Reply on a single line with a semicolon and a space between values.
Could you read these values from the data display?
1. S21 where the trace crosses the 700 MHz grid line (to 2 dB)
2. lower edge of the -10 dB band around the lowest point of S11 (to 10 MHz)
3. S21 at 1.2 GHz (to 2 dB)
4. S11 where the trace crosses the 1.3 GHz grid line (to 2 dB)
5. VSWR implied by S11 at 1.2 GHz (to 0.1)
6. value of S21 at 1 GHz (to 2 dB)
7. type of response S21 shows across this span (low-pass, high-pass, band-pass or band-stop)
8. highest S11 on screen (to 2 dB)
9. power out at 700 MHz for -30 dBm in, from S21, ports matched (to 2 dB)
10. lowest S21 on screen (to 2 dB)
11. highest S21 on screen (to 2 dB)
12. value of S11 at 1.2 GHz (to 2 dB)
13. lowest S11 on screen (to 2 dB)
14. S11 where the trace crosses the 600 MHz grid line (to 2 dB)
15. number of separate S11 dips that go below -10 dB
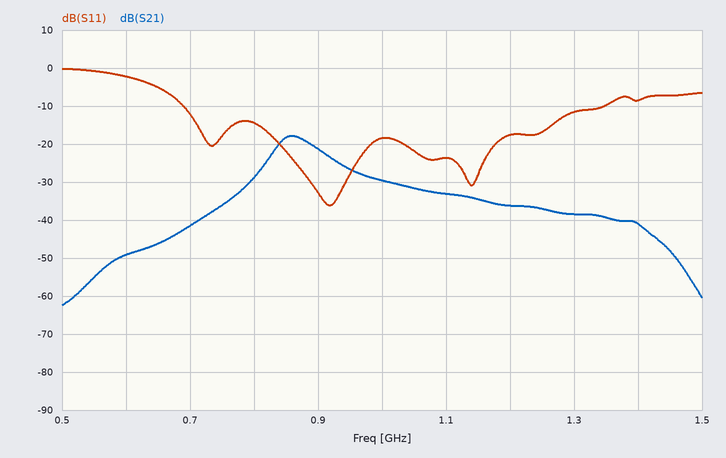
-42 dB; 690 MHz; -36 dB; -12 dB; 1.3; -30 dB; band-pass; 0 dB; -72 dBm; -62 dB; -18 dB; -18 dB; -36 dB; -2 dB; 3
